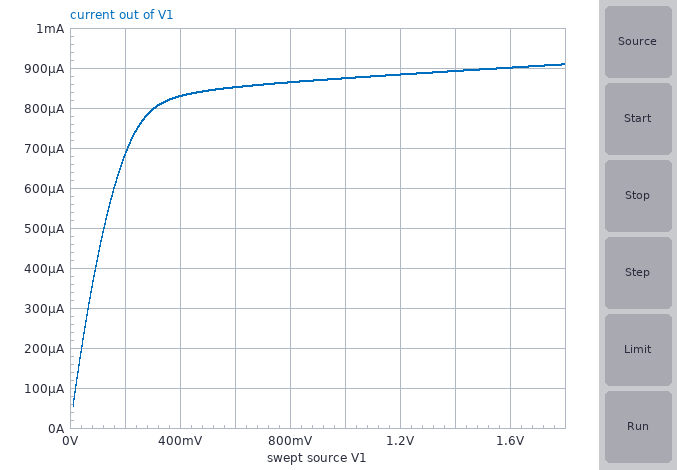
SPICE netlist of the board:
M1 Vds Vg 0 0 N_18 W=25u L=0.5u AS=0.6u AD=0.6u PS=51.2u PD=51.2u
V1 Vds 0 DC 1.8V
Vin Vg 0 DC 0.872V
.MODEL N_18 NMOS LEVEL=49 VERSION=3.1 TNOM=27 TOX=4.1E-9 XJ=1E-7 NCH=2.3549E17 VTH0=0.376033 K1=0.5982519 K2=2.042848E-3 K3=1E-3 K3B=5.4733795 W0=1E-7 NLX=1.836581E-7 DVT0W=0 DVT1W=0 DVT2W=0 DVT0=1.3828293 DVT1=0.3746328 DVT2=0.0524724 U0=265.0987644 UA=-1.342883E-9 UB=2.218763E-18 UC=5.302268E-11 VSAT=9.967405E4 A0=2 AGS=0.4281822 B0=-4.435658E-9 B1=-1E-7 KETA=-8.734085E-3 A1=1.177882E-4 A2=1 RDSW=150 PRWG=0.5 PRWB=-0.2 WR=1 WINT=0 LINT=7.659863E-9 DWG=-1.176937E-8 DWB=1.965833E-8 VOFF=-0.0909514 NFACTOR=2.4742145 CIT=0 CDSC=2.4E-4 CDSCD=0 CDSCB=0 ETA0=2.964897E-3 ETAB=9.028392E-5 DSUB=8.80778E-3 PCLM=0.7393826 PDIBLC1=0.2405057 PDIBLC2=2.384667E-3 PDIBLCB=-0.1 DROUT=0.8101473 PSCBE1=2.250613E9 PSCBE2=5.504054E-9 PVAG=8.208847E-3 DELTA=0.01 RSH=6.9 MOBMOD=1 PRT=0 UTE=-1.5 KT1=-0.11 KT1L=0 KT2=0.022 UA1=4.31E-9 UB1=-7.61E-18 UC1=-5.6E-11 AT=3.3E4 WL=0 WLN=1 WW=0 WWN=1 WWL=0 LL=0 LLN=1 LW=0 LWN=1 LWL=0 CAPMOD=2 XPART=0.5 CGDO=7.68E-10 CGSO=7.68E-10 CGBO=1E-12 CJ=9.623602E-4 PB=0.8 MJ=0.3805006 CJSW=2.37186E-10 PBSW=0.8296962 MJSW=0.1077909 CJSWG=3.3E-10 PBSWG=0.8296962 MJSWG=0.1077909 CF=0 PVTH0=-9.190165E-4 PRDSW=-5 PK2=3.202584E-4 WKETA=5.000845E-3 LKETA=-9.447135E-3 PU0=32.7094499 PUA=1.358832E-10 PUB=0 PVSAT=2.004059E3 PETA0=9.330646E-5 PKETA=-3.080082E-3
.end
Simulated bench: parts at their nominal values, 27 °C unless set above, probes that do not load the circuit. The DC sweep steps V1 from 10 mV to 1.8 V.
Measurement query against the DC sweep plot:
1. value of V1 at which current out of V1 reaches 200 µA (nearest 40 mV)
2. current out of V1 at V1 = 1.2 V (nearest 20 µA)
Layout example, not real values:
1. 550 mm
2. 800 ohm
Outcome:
1. 40 mV
2. 880 µA
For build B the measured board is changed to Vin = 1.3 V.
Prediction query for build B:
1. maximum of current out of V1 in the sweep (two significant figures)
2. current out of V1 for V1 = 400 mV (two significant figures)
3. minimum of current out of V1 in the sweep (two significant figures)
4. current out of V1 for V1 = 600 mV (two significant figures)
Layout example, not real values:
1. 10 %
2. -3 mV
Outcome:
1. 3.0 mA
2. 2.4 mA
3. 90 µA
4. 2.8 mA
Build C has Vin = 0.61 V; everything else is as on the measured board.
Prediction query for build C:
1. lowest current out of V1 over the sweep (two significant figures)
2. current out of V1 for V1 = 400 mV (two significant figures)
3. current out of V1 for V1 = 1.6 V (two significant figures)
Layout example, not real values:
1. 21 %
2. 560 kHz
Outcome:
1. 16 µA
2. 120 µA
3. 140 µA
